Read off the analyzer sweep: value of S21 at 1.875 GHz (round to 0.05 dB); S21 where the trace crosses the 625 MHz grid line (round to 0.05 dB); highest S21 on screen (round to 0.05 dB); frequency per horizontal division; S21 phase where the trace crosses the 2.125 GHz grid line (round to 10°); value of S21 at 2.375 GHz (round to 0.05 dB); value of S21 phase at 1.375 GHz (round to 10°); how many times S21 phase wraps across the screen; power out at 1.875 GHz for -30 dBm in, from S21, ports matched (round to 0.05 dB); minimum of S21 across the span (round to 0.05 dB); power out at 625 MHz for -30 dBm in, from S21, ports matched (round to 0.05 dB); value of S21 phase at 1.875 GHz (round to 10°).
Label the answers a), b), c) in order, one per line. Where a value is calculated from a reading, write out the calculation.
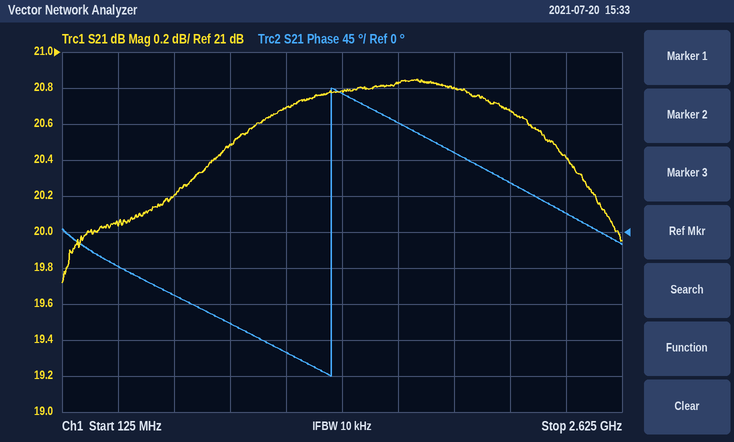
a) 20.80 dB
b) 20.20 dB
c) 20.85 dB
d) 250 MHz
e) 60°
f) 20.40 dB
g) 170°
h) 1
i) -30 dBm + (20.80 dB) = -9.20 dBm
j) 19.70 dB
k) -30 dBm + (20.20 dB) = -9.80 dBm
l) 100°
